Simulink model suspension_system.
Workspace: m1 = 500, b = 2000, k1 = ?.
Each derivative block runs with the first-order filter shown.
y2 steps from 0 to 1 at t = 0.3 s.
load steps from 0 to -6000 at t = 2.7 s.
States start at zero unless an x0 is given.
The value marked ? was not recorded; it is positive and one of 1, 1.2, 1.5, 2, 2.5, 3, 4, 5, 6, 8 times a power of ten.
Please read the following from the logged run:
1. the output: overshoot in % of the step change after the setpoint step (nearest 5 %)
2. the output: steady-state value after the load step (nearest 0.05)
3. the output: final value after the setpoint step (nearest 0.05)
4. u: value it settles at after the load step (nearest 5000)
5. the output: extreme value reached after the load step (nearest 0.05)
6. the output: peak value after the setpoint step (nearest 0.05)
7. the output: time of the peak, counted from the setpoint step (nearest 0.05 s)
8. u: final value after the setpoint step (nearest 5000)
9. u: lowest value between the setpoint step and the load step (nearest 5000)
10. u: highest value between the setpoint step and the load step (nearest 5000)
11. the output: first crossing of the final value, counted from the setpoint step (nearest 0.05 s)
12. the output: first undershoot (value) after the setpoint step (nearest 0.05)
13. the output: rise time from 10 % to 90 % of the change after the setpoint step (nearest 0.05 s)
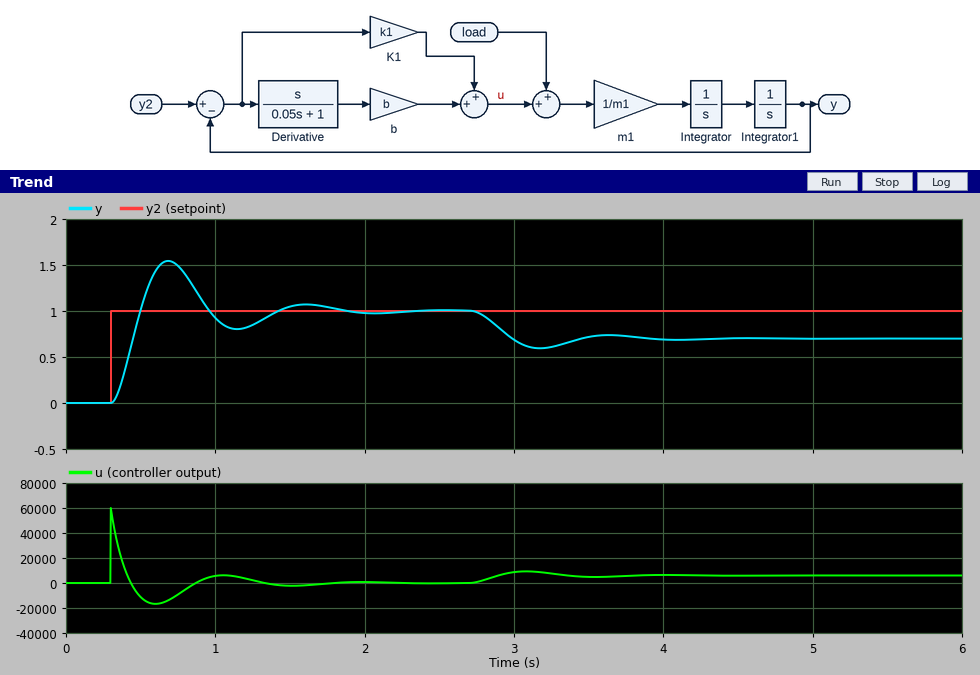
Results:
55 %
0.70
1.00
5000
0.60
1.55
0.40 s
0
-15000
60000
0.20 s
0.80
0.15 s
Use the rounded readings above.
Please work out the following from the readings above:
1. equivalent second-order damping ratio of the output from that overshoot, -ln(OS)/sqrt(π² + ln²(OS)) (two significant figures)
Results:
0.19
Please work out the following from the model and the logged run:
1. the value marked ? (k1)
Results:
20000
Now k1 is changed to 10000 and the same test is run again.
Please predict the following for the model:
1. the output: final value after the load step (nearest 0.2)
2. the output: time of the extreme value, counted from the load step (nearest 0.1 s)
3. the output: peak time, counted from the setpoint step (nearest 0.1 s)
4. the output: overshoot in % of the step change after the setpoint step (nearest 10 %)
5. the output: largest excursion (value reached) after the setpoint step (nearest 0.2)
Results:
0.4
0.7 s
0.5 s
40 %
1.4
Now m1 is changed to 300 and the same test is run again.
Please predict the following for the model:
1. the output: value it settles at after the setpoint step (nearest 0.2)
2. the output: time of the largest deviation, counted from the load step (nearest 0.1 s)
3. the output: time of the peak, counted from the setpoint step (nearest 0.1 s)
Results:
1.0
0.4 s
0.3 s
